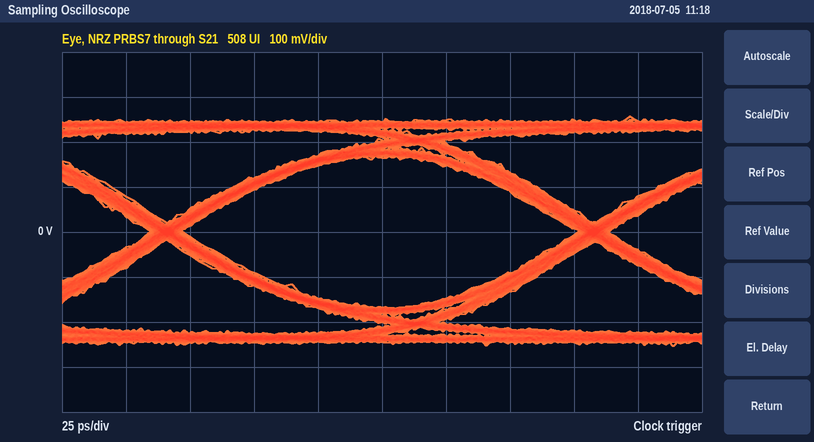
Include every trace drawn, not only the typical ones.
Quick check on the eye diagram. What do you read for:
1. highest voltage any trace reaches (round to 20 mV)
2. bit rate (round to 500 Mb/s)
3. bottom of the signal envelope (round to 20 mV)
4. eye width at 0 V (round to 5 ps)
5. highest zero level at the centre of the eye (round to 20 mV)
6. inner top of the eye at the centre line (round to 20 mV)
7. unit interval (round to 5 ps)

260 mV
6.0 Gb/s
-260 mV
155 ps
-160 mV
160 mV
165 ps
